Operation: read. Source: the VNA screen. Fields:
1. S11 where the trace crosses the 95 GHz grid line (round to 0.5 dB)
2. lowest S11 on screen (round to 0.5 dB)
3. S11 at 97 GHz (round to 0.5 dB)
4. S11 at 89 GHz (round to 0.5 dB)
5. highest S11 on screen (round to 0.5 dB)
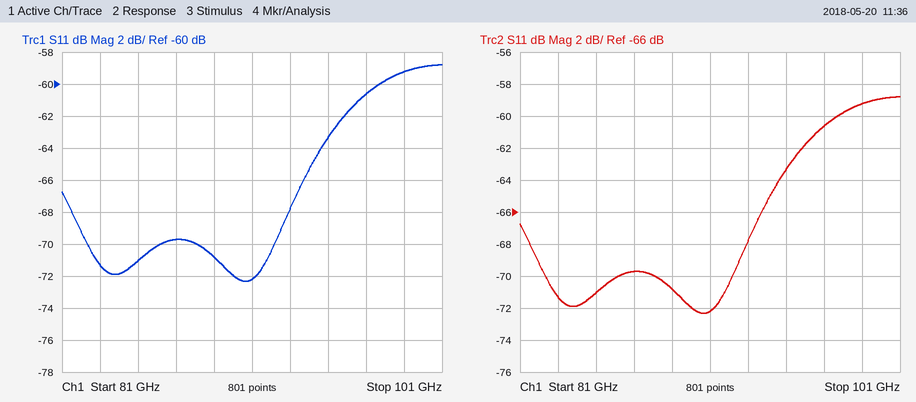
-63.5 dB
-72.5 dB
-60.5 dB
-71.0 dB
-59.0 dB
